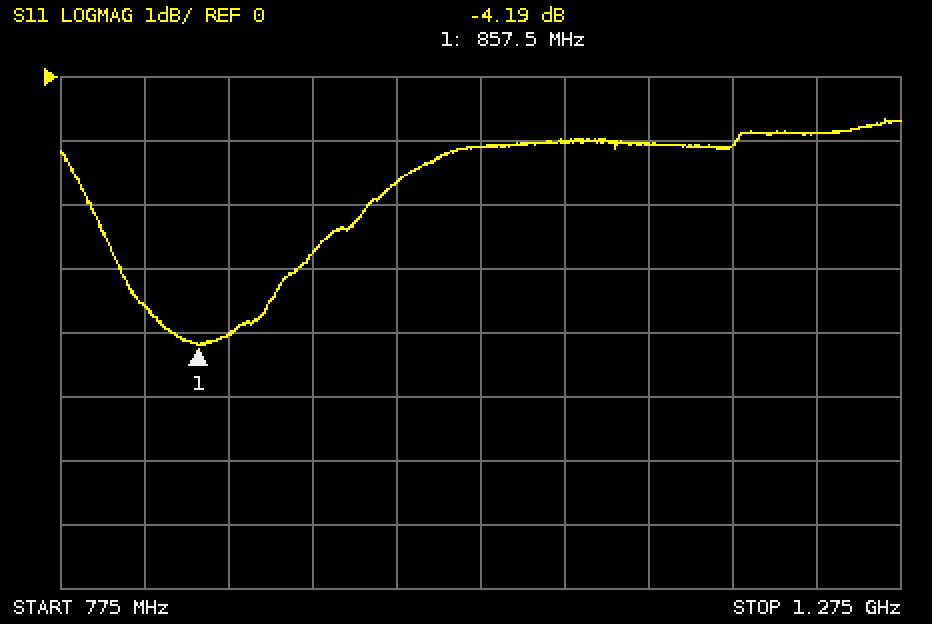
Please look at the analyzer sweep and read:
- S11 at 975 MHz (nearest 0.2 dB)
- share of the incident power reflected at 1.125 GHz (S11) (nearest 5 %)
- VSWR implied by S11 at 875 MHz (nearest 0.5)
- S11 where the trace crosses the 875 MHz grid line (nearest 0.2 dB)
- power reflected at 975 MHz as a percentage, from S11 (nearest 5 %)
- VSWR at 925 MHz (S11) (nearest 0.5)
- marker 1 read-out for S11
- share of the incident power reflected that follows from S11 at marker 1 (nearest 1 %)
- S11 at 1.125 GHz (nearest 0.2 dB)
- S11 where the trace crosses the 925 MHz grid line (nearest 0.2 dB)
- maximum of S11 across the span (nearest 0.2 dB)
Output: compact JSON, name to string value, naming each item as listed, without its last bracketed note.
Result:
{"S11 at 975 MHz": "-1.6 dB", "share of the incident power reflected at 1.125 GHz (S11)": "80 %", "VSWR implied by S11 at 875 MHz": "4.5", "S11 where the trace crosses the 875 MHz grid line": "-4.0 dB", "power reflected at 975 MHz as a percentage, from S11": "70 %", "VSWR at 925 MHz (S11)": "6.5", "marker 1 read-out for S11": "-4.19 dB", "share of the incident power reflected that follows from S11 at marker 1": "38 %", "S11 at 1.125 GHz": "-1.0 dB", "S11 where the trace crosses the 925 MHz grid line": "-2.8 dB", "maximum of S11 across the span": "-0.6 dB"}
